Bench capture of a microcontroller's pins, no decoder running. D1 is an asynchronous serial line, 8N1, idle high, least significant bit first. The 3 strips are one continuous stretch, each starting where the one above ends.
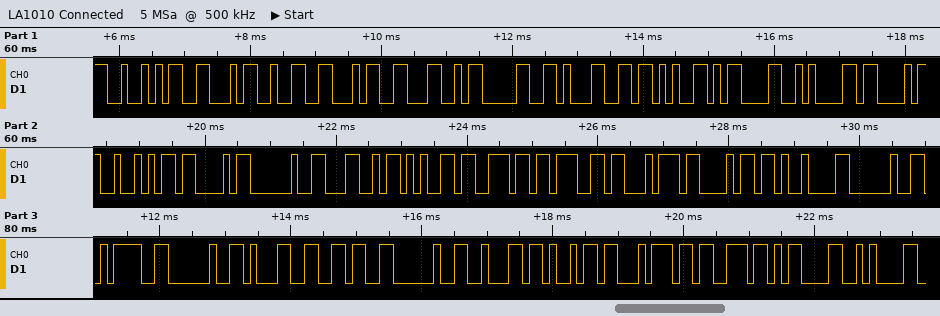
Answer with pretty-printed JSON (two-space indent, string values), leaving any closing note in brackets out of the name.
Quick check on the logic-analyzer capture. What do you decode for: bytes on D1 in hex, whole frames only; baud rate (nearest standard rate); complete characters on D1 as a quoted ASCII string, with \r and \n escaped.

{
  "bytes on D1 in hex, whole frames only": "0x52 0x46 0x32 0x34 0x4C 0x30 0x31 0x2B 0x0D 0x0A 0x43 0x52 0x43 0x20 0x4C 0x65 0x6E 0x67 0x74 0x68 0x09 0x20 0x3D 0x20 0x31 0x36 0x20 0x62 0x69 0x74 0x73 0x0D 0x0A",
  "baud rate": "9600 baud",
  "complete characters on D1 as a quoted ASCII string, with \\r and \\n escaped": "\"RF24L01+\\r\\nCRC Length\\t = 16 bits\\r\\n\""
}
